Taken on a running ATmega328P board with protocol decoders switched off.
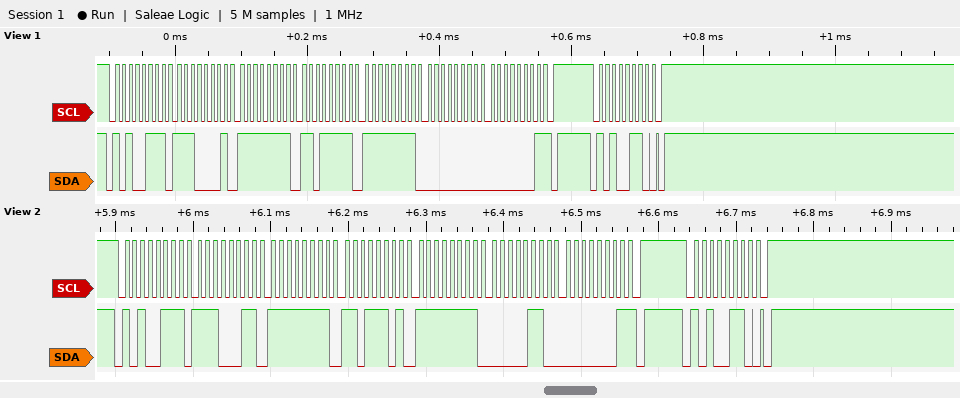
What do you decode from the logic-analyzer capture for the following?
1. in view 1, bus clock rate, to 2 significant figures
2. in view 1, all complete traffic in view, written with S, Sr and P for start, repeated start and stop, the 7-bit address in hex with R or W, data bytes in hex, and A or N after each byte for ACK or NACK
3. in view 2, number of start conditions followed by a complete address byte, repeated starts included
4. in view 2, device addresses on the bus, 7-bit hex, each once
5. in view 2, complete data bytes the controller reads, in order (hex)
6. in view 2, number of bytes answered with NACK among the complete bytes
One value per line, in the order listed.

100 kHz
S 53R A E1 A FF A DF A FF A 00 A 01 N P S 53W A P
2
0x53
E3 FF DD FF 06 01
1
